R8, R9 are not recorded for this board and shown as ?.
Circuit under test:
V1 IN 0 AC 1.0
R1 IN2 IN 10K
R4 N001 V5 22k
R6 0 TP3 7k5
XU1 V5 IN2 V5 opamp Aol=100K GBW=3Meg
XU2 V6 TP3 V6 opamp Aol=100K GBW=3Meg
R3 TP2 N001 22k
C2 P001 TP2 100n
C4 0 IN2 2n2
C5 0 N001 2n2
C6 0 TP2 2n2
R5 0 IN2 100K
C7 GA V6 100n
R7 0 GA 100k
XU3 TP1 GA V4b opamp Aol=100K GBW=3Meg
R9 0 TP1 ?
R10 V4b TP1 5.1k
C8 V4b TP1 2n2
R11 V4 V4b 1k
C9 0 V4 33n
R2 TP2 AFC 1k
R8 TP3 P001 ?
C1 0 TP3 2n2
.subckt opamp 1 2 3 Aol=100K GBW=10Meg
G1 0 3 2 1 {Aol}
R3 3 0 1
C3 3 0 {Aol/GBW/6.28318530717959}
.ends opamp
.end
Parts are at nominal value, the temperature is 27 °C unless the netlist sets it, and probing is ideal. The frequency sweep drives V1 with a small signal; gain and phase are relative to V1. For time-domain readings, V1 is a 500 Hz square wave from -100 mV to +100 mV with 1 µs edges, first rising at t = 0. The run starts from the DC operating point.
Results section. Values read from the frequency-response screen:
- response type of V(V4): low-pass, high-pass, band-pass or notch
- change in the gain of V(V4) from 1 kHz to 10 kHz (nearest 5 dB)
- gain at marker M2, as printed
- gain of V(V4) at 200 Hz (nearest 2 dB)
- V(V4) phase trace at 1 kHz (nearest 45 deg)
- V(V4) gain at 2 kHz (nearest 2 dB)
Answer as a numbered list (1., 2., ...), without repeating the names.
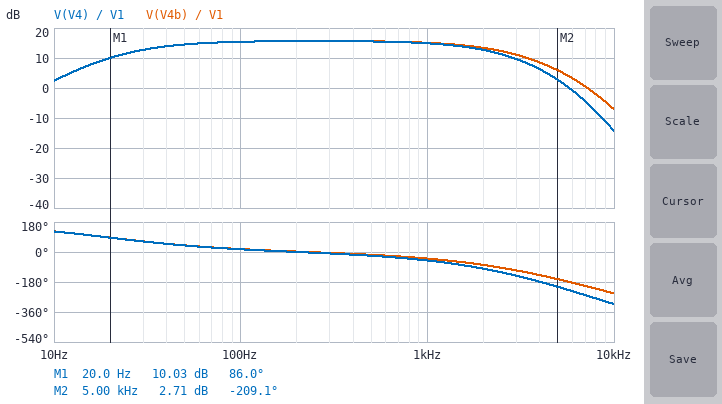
1. band-pass
2. -30 dB
3. 2.71 dB
4. 16 dB
5. -45 deg
6. 12 dB
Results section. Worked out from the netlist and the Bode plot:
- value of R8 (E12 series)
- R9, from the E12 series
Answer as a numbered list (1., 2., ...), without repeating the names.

1. 18 kΩ
2. 82 Ω
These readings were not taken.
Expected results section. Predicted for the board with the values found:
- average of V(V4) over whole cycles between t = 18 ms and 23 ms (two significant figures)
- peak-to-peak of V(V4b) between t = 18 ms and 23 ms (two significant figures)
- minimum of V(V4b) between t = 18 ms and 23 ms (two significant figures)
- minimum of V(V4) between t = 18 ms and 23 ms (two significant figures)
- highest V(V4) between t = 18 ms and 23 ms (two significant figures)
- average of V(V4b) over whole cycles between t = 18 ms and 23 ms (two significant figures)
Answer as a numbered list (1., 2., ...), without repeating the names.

1. -75 mV
2. 1.3 V
3. -720 mV
4. -720 mV
5. 570 mV
6. -75 mV
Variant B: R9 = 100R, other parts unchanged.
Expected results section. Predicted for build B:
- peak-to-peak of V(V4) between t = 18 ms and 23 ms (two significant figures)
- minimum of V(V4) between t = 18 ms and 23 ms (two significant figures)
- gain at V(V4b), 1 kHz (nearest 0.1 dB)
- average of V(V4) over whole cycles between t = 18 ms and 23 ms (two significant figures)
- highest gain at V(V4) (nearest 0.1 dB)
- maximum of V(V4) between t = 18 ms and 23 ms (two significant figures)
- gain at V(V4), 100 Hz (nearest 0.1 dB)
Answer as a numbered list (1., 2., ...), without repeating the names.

1. 1.1 V
2. -590 mV
3. 13.4 dB
4. -62 mV
5. 13.9 dB
6. 470 mV
7. 13.7 dB
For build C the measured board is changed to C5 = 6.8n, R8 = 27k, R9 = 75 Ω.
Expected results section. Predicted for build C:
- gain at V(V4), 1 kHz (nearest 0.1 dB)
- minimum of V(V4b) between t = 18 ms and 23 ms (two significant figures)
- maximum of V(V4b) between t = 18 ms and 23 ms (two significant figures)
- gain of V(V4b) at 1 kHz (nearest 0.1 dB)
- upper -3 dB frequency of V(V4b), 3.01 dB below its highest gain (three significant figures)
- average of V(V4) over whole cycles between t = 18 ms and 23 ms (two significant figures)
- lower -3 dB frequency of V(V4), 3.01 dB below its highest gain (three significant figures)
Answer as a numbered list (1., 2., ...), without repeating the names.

1. 12.9 dB
2. -660 mV
3. 510 mV
4. 13.1 dB
5. 1.22 kHz
6. -76 mV
7. 27.0 Hz
